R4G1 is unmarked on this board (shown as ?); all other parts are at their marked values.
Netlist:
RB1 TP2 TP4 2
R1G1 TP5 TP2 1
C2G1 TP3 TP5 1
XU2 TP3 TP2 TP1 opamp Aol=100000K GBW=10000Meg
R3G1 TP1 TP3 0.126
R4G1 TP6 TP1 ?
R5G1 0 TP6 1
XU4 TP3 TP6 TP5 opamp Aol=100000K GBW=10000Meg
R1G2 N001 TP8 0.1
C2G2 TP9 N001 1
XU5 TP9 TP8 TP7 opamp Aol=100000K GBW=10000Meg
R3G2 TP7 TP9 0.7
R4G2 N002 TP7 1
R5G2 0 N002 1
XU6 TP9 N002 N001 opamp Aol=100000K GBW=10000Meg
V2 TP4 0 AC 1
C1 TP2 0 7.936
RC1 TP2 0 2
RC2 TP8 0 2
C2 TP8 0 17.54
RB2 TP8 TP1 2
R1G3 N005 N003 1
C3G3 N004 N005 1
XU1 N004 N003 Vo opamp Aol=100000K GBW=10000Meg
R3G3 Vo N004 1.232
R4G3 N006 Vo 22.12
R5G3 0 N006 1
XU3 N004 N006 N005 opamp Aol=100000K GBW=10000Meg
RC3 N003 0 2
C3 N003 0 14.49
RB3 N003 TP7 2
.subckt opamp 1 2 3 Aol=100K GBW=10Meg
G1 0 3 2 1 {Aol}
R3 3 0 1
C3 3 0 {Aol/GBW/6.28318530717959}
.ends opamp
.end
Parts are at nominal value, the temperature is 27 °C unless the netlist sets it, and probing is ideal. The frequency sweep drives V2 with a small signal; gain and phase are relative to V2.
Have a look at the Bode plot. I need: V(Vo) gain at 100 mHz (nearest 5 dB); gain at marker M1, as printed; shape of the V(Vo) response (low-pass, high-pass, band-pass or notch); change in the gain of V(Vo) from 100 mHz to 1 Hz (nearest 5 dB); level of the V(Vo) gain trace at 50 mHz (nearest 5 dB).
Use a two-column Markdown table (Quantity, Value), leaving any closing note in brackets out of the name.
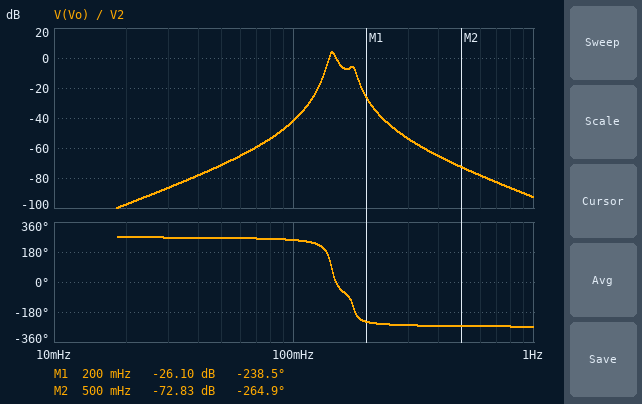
| Quantity | Value |
|---|---|
| V(Vo) gain at 100 mHz | -40 dB |
| gain at marker M1, as printed | -26.10 dB |
| shape of the V(Vo) response | band-pass |
| change in the gain of V(Vo) from 100 mHz to 1 Hz | -50 dB |
| level of the V(Vo) gain trace at 50 mHz | -70 dB |
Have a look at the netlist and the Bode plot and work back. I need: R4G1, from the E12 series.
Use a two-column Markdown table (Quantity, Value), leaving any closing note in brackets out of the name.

| Quantity | Value |
|---|---|
| R4G1, from the E12 series | 0.82 Ω |
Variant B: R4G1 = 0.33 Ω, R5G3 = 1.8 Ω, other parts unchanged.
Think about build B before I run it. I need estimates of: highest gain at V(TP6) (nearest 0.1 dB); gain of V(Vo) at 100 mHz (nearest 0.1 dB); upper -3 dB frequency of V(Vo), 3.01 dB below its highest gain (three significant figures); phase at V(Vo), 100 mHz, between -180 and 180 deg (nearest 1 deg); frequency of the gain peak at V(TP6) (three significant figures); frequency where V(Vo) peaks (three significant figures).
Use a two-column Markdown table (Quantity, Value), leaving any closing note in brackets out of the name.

| Quantity | Value |
|---|---|
| highest gain at V(TP6) | -6.0 dB |
| gain of V(Vo) at 100 mHz | -27.4 dB |
| upper -3 dB frequency of V(Vo), 3.01 dB below its highest gain | 146 mHz |
| phase at V(Vo), 100 mHz, between -180 and 180 deg | 127 deg |
| frequency of the gain peak at V(TP6) | 91.4 mHz |
| frequency where V(Vo) peaks | 141 mHz |
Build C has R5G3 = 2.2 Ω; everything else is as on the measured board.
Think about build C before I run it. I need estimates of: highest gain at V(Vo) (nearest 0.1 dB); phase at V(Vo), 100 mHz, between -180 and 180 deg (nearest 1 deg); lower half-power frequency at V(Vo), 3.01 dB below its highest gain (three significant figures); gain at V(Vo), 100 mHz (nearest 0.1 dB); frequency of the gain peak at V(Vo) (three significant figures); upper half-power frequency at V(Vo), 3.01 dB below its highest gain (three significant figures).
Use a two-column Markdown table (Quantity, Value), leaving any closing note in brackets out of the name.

| Quantity | Value |
|---|---|
| highest gain at V(Vo) | 1.7 dB |
| phase at V(Vo), 100 mHz, between -180 and 180 deg | -120 deg |
| lower half-power frequency at V(Vo), 3.01 dB below its highest gain | 139 mHz |
| gain at V(Vo), 100 mHz | -34.2 dB |
| frequency of the gain peak at V(Vo) | 143 mHz |
| upper half-power frequency at V(Vo), 3.01 dB below its highest gain | 147 mHz |
